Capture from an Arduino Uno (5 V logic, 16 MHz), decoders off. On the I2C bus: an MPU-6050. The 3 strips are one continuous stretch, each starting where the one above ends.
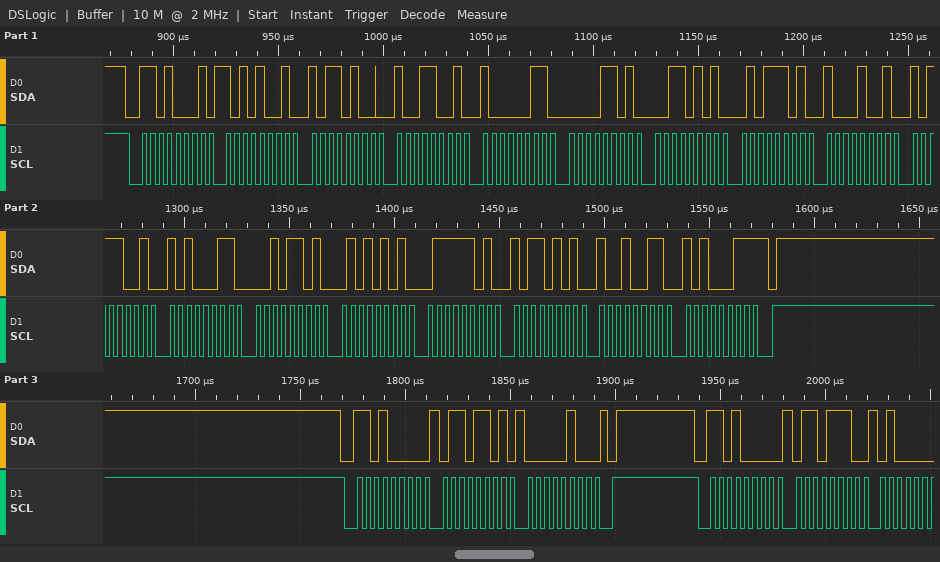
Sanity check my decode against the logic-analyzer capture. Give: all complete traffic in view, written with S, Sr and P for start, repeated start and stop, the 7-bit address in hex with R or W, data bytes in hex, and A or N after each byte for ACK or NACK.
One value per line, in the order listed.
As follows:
S 68R A A9 A B4 A 99 A 83 A 0D A 35 A 5D A 89 A B9 A A3 A 2D A 55 A 7D A B5 A 93 A A3 N P S 68W A 6D A 04 A P S 68W A 6E A
